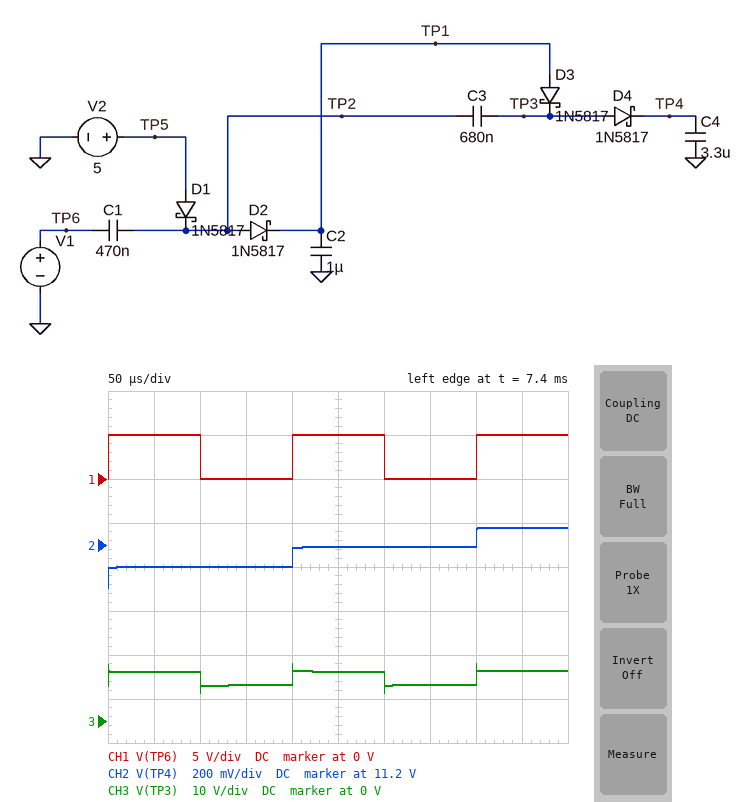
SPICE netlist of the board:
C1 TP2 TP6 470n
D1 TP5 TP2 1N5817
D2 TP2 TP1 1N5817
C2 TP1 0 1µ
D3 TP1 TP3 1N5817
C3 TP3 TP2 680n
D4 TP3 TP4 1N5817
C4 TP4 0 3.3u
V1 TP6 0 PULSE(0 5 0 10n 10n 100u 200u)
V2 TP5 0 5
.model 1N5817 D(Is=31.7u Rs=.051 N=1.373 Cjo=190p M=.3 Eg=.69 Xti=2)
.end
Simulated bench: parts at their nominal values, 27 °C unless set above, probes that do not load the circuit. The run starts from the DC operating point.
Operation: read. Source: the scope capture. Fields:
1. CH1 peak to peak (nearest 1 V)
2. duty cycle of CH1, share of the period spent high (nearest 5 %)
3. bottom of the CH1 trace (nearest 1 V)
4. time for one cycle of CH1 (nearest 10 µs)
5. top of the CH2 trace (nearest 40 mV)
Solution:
5 V
50 %
0 V
200 µs
11.28 V
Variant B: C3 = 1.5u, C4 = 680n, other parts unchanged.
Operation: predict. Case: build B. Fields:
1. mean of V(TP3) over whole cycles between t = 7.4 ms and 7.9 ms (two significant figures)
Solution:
12 V
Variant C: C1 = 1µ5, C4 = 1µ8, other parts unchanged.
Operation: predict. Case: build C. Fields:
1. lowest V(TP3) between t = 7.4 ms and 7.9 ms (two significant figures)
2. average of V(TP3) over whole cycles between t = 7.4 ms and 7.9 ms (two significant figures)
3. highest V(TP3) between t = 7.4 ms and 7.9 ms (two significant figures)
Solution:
9.5 V
12 V
15 V
